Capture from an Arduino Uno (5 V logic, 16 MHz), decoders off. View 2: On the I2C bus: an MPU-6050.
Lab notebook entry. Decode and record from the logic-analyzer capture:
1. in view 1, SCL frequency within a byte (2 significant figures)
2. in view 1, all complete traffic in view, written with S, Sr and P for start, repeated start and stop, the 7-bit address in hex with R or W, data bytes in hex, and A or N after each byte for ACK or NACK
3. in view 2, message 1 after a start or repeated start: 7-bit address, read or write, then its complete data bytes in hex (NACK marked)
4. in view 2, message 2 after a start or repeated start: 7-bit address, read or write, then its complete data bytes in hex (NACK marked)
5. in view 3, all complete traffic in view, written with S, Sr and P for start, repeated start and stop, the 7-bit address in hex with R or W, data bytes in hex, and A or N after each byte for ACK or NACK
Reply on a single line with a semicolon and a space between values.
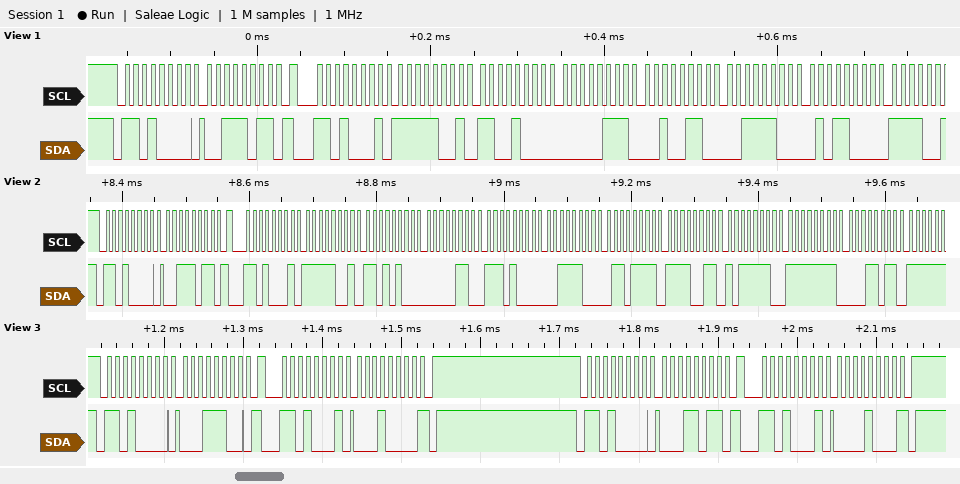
100 kHz; S 68W A 3B A Sr 68R A F9 A C8 A 07 A 26 A 3C A 58 A; 0x68 write: 3B; 0x68 read: F9 D4 06 E8 3C 6F F3 BE FF 1B; S 68W A 1C A Sr 68R A 10 N P S 68W A 1B A Sr 68R A 08 N P
